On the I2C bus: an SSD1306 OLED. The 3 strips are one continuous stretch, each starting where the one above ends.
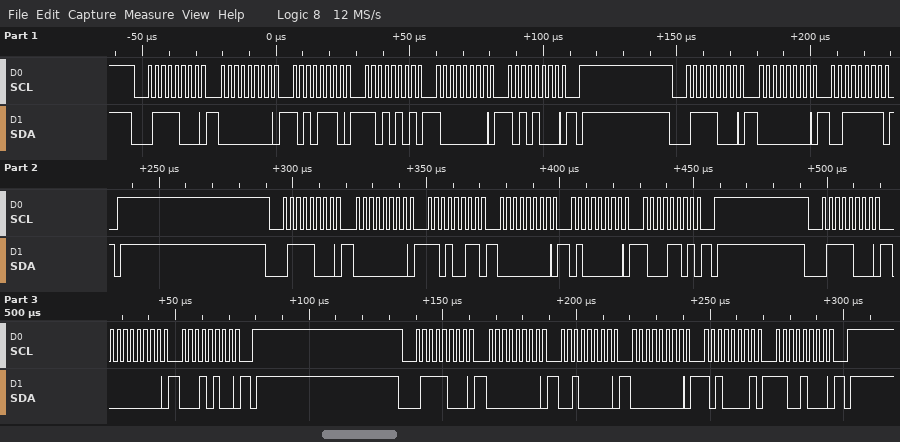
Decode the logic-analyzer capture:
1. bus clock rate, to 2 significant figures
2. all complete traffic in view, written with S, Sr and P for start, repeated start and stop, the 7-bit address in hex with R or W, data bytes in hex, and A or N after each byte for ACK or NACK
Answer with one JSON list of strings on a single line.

["400 kHz", "S 3CW A 00 A AE A D5 A 80 A A8 A P S 3CW A 00 A 3F A P S 3CW A 00 A D3 A 00 A 40 A 8D A P S 3CW A 00 A 14 A P S 3CW A 00 A 20 A 00 A A1 A C8 A P"]
